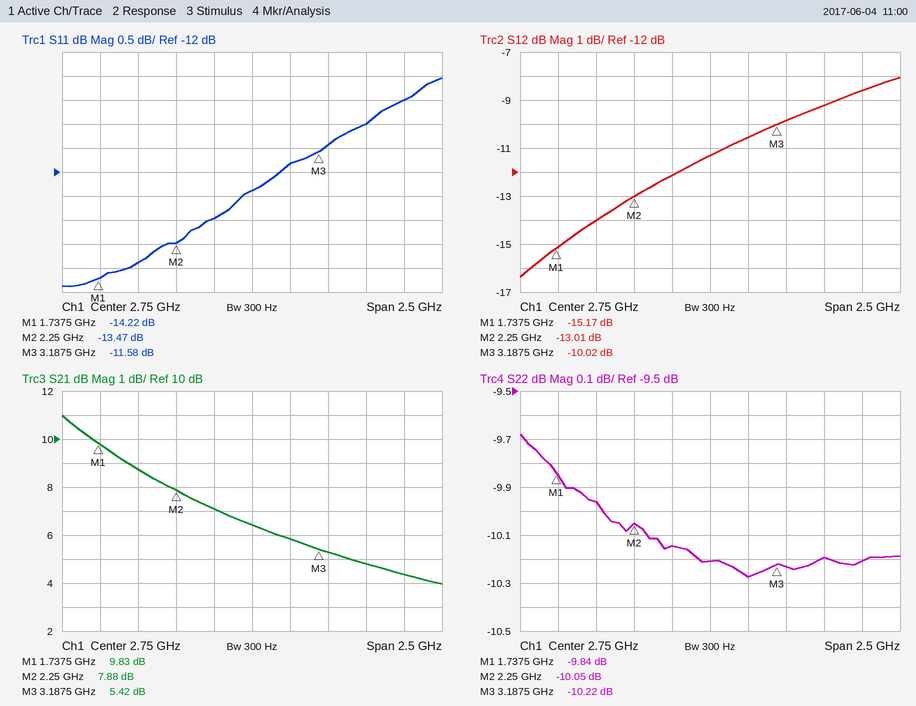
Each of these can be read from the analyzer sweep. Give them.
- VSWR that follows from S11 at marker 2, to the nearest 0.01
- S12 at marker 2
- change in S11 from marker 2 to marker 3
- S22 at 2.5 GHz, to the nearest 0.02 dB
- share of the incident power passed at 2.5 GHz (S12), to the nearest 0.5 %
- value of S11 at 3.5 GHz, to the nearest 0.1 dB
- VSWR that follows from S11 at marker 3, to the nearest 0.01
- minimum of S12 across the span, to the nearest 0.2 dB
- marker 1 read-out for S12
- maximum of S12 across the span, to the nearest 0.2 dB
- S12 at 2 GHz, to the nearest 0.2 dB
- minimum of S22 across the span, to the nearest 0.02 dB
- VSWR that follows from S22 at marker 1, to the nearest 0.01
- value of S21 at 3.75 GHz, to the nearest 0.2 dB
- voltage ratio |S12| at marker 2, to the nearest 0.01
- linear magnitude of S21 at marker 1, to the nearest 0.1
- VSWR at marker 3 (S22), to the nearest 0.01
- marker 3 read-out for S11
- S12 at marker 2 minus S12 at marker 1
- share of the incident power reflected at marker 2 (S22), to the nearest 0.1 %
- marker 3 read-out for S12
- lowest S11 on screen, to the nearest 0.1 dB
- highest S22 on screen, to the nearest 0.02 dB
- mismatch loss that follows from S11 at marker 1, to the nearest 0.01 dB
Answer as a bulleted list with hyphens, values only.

- 1.54
- -13.01 dB
- 1.89 dB
- -10.14 dB
- 6.0 %
- -11.0 dB
- 1.72
- -16.4 dB
- -15.17 dB
- -8.0 dB
- -14.0 dB
- -10.28 dB
- 1.95
- 4.4 dB
- 0.22
- 3.1
- 1.89
- -11.58 dB
- 2.16 dB
- 9.9 %
- -10.02 dB
- -14.4 dB
- -9.68 dB
- 0.17 dB
